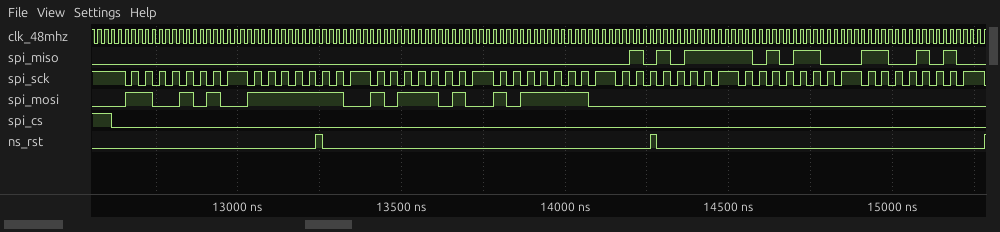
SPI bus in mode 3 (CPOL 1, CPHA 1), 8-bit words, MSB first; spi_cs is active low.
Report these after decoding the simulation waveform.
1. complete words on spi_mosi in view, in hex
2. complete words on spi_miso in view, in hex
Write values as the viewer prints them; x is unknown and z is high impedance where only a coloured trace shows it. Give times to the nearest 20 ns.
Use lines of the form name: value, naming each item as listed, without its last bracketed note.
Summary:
complete words on spi_mosi in view, in hex: CA, FE, BA, BE, 00, 00, 00
complete words on spi_miso in view, in hex: 00, 00, 00, 00, 57, AC, CA
